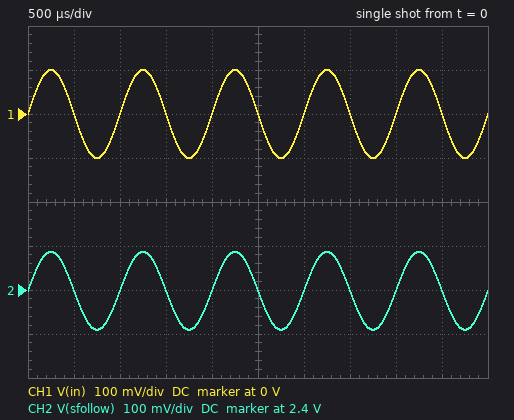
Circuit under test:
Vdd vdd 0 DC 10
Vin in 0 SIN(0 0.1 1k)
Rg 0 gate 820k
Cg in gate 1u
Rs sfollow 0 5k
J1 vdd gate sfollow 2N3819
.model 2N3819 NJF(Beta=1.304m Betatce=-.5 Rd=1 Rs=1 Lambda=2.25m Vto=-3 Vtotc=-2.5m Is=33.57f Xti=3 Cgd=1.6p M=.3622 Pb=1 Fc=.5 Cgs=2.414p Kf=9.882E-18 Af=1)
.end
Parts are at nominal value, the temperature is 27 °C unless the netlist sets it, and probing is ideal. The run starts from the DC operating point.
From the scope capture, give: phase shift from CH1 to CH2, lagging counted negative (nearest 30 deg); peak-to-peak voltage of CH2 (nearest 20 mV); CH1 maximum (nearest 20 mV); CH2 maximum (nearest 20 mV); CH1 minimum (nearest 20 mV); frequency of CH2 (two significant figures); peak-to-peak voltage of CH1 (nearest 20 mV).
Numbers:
0 deg
180 mV
100 mV
2.48 V
-100 mV
1.0 kHz
200 mV
